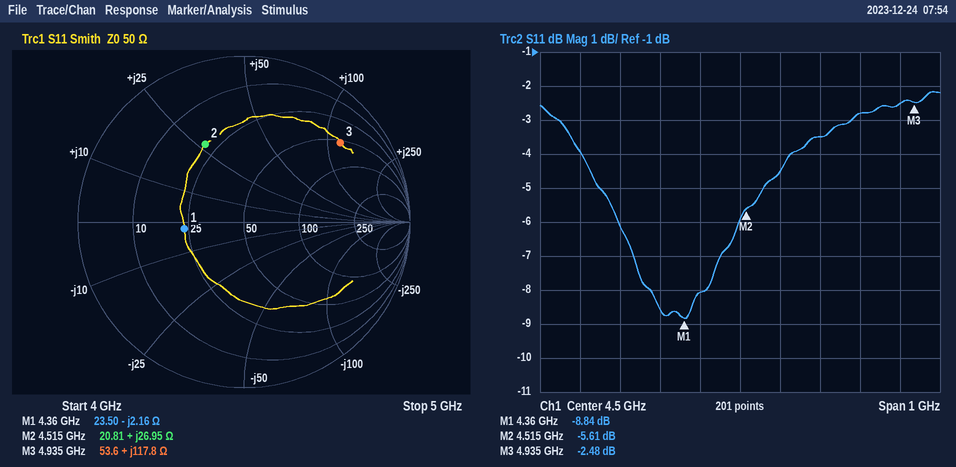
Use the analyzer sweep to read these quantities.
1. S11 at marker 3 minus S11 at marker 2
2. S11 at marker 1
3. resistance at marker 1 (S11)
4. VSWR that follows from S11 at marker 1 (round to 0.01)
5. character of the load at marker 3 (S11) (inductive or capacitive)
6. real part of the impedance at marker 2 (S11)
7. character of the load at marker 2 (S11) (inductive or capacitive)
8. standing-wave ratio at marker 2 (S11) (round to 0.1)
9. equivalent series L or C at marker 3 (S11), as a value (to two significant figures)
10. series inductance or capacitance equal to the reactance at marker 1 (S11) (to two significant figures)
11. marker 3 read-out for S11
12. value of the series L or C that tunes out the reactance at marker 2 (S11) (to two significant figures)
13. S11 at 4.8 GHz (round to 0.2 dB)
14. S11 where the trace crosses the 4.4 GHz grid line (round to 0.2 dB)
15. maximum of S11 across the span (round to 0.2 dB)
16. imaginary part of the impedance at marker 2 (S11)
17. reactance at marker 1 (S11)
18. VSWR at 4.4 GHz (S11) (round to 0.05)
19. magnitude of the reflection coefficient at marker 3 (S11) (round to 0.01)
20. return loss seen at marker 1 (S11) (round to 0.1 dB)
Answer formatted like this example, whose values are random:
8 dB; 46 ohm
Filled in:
3.13 dB; -8.84 dB; 23.50 Ω; 2.13; inductive; 20.81 Ω; inductive; 3.2; 3.8 nH; 17 pF; -2.48 dB; 1.3 pF; -2.8 dB; -8.0 dB; -2.2 dB; +26.95 Ω; -2.16 Ω; 2.30; 0.75; 8.8 dB
